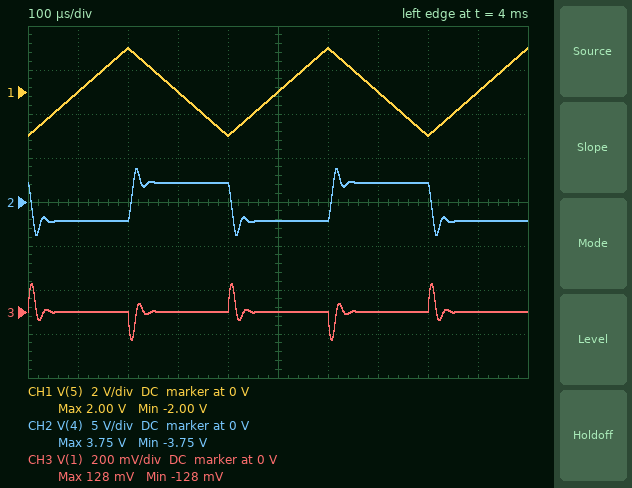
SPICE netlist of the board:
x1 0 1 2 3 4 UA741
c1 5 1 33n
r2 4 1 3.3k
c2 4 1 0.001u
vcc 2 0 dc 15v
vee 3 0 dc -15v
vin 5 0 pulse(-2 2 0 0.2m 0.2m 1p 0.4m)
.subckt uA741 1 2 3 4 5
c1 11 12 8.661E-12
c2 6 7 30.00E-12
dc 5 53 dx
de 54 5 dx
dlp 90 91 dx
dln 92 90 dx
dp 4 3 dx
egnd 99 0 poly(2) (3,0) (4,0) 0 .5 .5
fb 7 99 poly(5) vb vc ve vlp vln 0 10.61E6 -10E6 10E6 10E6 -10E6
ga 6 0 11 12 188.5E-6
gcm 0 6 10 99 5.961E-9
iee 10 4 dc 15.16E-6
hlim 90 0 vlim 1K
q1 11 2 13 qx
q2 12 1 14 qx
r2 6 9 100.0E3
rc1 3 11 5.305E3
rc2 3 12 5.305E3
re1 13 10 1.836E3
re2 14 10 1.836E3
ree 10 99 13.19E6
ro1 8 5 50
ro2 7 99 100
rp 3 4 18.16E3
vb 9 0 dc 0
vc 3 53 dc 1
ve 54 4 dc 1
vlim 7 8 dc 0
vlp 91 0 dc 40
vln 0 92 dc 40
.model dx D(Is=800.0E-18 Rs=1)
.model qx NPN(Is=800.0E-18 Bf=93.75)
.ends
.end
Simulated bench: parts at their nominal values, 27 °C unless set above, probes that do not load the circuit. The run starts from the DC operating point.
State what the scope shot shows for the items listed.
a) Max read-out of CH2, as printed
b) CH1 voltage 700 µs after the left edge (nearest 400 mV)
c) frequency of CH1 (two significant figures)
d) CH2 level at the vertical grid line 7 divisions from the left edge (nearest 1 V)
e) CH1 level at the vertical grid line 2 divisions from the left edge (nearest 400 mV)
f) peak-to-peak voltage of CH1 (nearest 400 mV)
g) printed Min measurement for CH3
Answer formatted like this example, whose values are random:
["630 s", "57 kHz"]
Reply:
["3.75 V", "0 V", "2.5 kHz", "2 V", "2.0 V", "4.0 V", "-128 mV"]
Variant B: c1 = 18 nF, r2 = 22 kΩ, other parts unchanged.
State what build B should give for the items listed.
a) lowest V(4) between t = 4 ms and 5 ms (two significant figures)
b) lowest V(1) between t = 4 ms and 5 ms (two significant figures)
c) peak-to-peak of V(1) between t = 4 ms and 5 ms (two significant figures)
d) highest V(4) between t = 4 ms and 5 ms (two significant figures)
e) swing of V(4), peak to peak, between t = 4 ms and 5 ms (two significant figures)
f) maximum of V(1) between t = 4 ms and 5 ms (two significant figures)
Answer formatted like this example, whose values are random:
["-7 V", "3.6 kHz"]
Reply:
["-7.9 V", "-140 mV", "280 mV", "7.9 V", "16 V", "140 mV"]
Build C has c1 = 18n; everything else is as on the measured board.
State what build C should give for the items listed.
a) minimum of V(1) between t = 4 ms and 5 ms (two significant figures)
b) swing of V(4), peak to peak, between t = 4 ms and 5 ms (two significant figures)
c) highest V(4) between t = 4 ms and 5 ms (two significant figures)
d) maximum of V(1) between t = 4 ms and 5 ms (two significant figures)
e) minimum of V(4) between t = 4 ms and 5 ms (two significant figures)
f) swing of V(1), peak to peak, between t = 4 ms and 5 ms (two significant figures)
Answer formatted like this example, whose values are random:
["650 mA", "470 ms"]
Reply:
["-72 mV", "3.2 V", "1.6 V", "72 mV", "-1.6 V", "140 mV"]
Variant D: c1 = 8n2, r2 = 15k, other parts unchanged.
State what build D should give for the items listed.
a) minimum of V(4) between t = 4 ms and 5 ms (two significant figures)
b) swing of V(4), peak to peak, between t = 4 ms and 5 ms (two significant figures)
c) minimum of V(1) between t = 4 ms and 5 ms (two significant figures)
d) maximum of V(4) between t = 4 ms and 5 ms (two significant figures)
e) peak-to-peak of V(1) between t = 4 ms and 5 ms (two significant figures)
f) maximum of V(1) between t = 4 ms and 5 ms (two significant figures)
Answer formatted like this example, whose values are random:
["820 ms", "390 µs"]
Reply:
["-2.5 V", "4.9 V", "-47 mV", "2.5 V", "94 mV", "47 mV"]
